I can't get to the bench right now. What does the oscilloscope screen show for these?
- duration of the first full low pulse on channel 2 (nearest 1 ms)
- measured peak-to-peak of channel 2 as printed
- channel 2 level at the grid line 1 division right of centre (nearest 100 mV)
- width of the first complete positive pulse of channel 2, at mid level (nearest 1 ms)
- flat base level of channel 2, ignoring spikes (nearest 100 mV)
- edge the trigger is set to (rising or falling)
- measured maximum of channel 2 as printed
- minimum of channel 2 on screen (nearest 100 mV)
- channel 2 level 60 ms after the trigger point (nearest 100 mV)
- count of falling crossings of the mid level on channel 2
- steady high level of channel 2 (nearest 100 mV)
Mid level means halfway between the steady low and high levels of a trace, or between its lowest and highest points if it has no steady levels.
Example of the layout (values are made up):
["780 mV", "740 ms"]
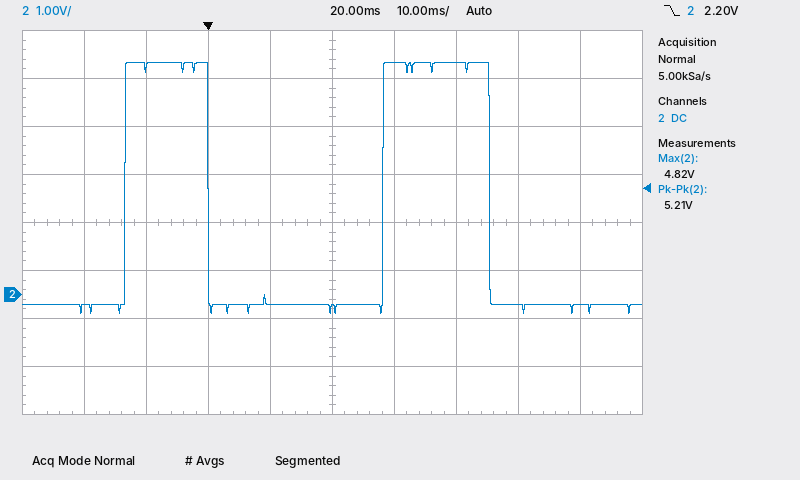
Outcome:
["28 ms", "5.21 V", "4.8 V", "13 ms", "-200 mV", "falling", "4.82 V", "-400 mV", "-200 mV", "2", "4.8 V"]
